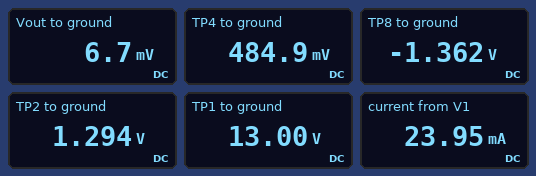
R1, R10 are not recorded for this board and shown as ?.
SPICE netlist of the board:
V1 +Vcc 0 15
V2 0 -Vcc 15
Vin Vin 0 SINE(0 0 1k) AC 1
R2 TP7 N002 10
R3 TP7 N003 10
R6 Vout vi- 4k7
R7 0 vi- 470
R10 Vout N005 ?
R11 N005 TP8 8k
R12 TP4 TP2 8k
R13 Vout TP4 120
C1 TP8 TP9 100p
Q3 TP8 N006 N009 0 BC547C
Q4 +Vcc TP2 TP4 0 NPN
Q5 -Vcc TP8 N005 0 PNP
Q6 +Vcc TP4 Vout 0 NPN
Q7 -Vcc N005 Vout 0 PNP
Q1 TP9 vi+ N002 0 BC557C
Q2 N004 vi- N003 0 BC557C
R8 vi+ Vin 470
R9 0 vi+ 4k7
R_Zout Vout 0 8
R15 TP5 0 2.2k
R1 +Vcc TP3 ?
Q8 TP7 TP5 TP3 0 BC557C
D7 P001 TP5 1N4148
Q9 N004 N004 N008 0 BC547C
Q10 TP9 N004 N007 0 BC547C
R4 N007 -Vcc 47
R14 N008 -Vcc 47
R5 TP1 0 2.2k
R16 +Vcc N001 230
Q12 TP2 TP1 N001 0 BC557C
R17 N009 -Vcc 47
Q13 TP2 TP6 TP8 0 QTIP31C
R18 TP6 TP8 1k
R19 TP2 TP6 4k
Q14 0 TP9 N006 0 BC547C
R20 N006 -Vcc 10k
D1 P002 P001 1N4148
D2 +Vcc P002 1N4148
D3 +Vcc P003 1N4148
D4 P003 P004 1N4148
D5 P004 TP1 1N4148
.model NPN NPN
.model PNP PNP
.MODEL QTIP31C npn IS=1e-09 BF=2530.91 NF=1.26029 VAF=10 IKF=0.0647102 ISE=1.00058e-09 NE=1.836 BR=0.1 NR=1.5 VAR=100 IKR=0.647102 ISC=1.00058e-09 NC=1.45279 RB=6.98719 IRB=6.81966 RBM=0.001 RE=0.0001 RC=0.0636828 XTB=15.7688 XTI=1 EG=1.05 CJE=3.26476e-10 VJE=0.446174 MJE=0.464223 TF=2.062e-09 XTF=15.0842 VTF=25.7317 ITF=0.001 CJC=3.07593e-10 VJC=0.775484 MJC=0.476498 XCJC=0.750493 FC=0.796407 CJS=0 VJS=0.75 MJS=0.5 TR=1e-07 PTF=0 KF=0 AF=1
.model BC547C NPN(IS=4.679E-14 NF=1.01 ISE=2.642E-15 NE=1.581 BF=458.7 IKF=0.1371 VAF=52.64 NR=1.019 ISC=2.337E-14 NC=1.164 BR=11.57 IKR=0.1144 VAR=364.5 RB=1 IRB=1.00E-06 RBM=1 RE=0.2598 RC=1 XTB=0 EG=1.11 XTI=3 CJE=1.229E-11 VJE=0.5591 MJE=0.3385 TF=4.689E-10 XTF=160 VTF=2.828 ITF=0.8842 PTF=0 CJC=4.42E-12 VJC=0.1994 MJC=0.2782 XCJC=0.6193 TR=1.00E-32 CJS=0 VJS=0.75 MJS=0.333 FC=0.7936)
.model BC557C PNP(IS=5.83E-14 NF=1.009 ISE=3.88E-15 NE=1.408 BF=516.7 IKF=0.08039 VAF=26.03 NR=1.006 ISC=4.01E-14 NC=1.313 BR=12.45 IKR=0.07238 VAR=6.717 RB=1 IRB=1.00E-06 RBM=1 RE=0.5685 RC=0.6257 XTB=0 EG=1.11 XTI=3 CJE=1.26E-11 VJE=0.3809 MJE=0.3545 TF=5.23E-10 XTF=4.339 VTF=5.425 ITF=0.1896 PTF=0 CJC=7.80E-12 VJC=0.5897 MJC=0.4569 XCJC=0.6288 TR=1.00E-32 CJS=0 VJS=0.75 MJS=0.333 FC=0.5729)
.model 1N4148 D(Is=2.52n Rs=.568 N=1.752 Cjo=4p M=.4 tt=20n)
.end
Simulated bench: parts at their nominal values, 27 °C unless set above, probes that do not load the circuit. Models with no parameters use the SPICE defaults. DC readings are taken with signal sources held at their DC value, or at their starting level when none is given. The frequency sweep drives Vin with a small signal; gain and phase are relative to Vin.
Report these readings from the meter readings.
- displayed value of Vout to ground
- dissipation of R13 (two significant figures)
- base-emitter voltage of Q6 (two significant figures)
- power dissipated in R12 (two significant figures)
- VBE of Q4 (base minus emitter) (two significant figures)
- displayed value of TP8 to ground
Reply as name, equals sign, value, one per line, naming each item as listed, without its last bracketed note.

displayed value of Vout to ground = 6.7 mV
dissipation of R13 = 1.9 mW
base-emitter voltage of Q6 = 480 mV
power dissipated in R12 = 82 µW
VBE of Q4 (base minus emitter) = 810 mV
displayed value of TP8 to ground = -1.362 V
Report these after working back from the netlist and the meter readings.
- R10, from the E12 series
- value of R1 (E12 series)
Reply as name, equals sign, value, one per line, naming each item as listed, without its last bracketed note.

R10, from the E12 series = 180 Ω
value of R1 = 560 Ω
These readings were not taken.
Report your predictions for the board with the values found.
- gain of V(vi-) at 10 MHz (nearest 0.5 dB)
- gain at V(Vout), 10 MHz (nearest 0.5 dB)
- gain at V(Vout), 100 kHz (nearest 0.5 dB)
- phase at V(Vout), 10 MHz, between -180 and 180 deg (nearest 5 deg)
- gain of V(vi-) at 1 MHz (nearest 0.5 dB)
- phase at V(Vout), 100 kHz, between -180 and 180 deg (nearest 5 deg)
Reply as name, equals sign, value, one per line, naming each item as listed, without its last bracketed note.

gain of V(vi-) at 10 MHz = -10.5 dB
gain at V(Vout), 10 MHz = -10.5 dB
gain at V(Vout), 100 kHz = 20.0 dB
phase at V(Vout), 10 MHz, between -180 and 180 deg = -170 deg
gain of V(vi-) at 1 MHz = -10.0 dB
phase at V(Vout), 100 kHz, between -180 and 180 deg = -15 deg
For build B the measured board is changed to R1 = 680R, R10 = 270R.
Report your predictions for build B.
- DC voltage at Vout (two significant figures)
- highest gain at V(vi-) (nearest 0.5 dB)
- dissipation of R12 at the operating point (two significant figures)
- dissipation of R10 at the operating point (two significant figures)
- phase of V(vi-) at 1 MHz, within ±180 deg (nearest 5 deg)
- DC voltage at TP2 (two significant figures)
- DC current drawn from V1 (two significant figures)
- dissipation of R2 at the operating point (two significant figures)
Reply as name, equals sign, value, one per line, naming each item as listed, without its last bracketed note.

DC voltage at Vout = 7.1 mV
highest gain at V(vi-) = -1.0 dB
dissipation of R12 at the operating point = 81 µW
dissipation of R10 at the operating point = 1.6 mW
phase of V(vi-) at 1 MHz, within ±180 deg = -80 deg
DC voltage at TP2 = 1.2 V
DC current drawn from V1 = 23 mA
dissipation of R2 at the operating point = 10 µW
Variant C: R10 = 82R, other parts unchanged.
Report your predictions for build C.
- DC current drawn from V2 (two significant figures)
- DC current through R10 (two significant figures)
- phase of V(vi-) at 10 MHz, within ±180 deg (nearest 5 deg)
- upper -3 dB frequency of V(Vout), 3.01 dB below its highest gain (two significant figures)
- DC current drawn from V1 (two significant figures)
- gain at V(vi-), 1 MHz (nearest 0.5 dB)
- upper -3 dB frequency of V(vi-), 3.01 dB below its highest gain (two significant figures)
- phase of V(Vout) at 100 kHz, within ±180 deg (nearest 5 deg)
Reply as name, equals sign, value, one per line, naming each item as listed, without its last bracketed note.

DC current drawn from V2 = 13 mA
DC current through R10 = 4.6 mA
phase of V(vi-) at 10 MHz, within ±180 deg = 40 deg
upper -3 dB frequency of V(Vout), 3.01 dB below its highest gain = 650 kHz
DC current drawn from V1 = 25 mA
gain at V(vi-), 1 MHz = -7.0 dB
upper -3 dB frequency of V(vi-), 3.01 dB below its highest gain = 610 kHz
phase of V(Vout) at 100 kHz, within ±180 deg = -10 deg
